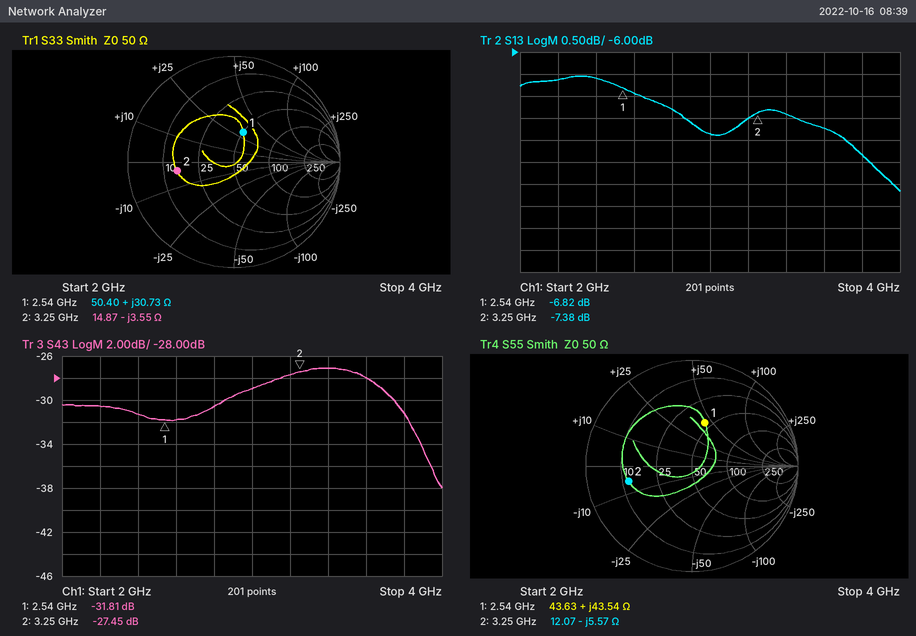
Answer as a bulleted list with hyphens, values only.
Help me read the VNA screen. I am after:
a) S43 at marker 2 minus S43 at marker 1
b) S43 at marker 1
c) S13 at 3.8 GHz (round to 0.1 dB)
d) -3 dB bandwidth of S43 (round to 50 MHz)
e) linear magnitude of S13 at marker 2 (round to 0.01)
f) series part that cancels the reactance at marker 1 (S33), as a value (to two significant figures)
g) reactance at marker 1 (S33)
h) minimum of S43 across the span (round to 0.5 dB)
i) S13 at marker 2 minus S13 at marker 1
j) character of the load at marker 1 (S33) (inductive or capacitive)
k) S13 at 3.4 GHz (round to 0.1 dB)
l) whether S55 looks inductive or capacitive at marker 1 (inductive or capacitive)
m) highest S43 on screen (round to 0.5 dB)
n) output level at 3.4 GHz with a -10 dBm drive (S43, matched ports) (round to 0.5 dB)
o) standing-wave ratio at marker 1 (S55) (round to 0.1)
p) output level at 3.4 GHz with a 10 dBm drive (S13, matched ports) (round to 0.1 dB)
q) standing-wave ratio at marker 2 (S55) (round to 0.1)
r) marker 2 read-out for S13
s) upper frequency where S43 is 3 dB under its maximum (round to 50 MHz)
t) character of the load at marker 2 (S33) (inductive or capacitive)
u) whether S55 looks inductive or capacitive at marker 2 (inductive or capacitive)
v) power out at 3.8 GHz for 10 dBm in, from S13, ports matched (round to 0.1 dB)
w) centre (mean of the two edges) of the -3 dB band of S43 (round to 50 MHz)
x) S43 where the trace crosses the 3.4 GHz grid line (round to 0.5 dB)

- 4.36 dB
- -31.81 dB
- -8.3 dB
- 900 MHz
- 0.43
- 2.0 pF
- +30.73 Ω
- -38.0 dB
- -0.56 dB
- inductive
- -7.4 dB
- inductive
- -27.0 dB
- -37.0 dBm
- 2.5
- 2.6 dBm
- 4.2
- -7.38 dB
- 3.75 GHz
- capacitive
- capacitive
- 1.7 dBm
- 3.30 GHz
- -27.0 dB
